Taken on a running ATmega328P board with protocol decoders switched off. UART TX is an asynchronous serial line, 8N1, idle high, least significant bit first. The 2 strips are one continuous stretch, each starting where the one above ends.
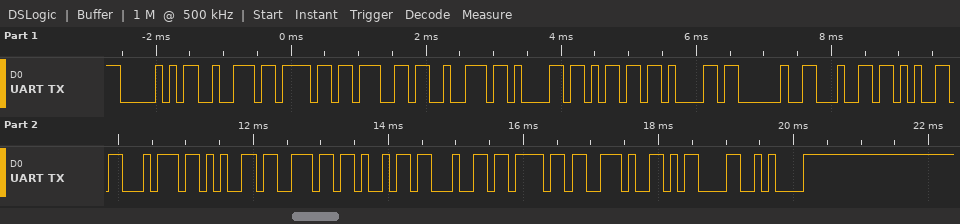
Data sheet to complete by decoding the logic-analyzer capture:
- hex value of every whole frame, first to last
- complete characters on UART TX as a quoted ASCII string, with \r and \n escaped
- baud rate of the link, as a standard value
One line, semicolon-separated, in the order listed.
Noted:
50 72 6F 67 72 61 6D 61 20 64 65 74 65 6E 69 64 6F 2E 0D 0A; "Programa detenido.\r\n"; 9600 baud
